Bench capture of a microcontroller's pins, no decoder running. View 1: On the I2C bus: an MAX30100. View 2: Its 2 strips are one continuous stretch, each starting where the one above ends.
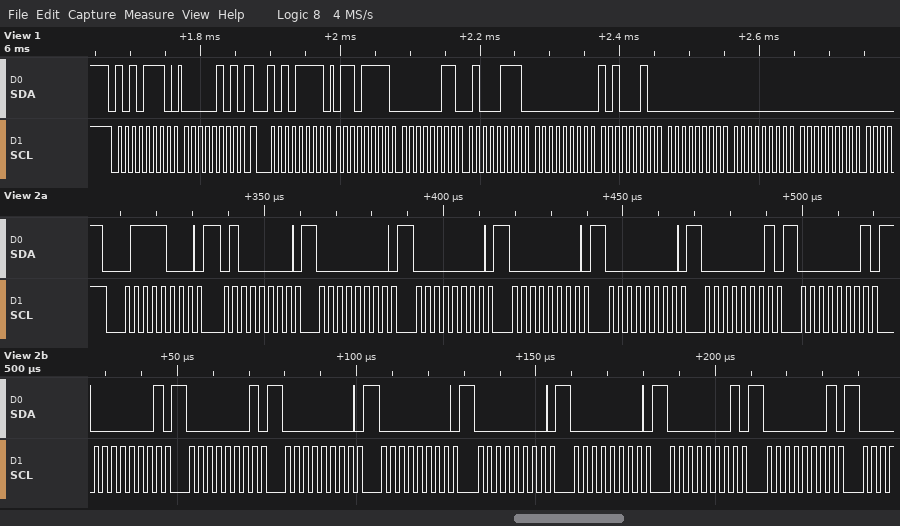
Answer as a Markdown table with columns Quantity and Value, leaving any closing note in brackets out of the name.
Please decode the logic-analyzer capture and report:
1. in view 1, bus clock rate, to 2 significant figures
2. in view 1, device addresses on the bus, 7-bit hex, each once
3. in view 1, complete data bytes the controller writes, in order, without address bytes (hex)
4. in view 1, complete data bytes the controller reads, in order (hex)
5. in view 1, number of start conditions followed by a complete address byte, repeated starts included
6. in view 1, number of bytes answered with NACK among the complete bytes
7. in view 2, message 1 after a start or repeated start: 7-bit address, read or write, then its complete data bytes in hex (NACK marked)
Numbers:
| Quantity | Value |
|---|---|
| in view 1, bus clock rate, to 2 significant figures | 100 kHz |
| in view 1, device addresses on the bus, 7-bit hex, each once | 0x57 |
| in view 1, complete data bytes the controller writes, in order, without address bytes | 05 |
| in view 1, complete data bytes the controller reads, in order | 6F 03 47 00 A2 00 00 00 |
| in view 1, number of start conditions followed by a complete address byte, repeated starts included | 2 |
| in view 1, number of bytes answered with NACK among the complete bytes | 0 |
| in view 2, message 1 after a start or repeated start: 7-bit address, read or write, then its complete data bytes in hex | 0x3C write: 40 00 00 00 00 01 01 01 01 00 00 00 00 01 01 |
